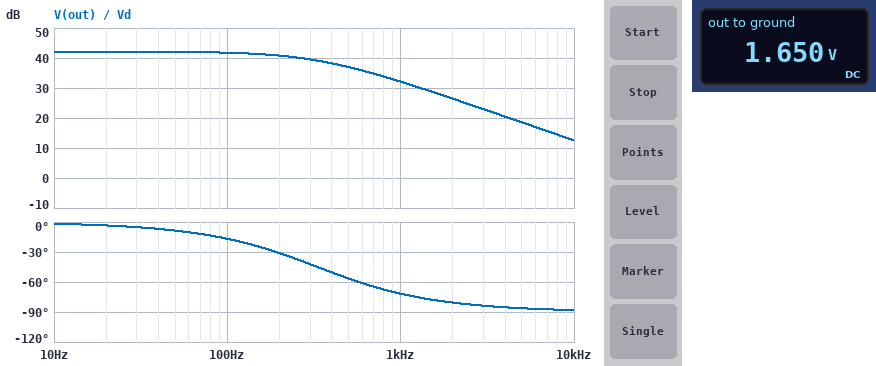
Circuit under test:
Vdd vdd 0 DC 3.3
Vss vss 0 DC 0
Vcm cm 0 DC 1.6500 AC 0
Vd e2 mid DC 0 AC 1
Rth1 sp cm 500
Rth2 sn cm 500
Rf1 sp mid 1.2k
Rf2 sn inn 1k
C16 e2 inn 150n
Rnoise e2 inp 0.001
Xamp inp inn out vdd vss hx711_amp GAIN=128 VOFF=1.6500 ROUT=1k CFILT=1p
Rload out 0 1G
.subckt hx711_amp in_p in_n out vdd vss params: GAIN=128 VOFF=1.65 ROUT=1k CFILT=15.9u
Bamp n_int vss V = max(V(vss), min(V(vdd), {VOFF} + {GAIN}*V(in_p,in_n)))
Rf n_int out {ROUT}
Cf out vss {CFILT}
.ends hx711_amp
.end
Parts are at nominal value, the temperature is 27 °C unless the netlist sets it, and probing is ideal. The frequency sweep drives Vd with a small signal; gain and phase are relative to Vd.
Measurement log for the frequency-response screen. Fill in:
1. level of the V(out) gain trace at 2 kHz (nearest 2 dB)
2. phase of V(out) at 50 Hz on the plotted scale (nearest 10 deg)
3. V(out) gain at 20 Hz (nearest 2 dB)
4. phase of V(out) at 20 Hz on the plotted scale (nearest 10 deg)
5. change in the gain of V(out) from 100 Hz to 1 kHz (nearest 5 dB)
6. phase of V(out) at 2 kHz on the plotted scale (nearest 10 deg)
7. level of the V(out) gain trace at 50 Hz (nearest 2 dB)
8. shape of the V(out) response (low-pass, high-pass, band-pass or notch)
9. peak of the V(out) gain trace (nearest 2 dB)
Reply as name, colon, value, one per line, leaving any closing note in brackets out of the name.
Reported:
level of the V(out) gain trace at 2 kHz: 26 dB
phase of V(out) at 50 Hz on the plotted scale: -10 deg
V(out) gain at 20 Hz: 42 dB
phase of V(out) at 20 Hz on the plotted scale: 0 deg
change in the gain of V(out) from 100 Hz to 1 kHz: -10 dB
phase of V(out) at 2 kHz on the plotted scale: -80 deg
level of the V(out) gain trace at 50 Hz: 42 dB
shape of the V(out) response: low-pass
peak of the V(out) gain trace: 42 dB
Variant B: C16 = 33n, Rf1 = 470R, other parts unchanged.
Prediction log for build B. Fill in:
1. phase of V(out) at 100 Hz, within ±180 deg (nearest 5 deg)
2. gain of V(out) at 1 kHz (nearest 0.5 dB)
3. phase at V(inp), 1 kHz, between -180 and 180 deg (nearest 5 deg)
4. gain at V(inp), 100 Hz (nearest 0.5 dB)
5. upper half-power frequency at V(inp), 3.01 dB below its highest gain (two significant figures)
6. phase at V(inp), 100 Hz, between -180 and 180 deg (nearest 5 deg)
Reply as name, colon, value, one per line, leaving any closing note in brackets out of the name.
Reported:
phase of V(out) at 100 Hz, within ±180 deg: -5 deg
gain of V(out) at 1 kHz: 41.0 dB
phase at V(inp), 1 kHz, between -180 and 180 deg: -10 deg
gain at V(inp), 100 Hz: 0 dB
upper half-power frequency at V(inp), 3.01 dB below its highest gain: 3.8 kHz
phase at V(inp), 100 Hz, between -180 and 180 deg: 0 deg
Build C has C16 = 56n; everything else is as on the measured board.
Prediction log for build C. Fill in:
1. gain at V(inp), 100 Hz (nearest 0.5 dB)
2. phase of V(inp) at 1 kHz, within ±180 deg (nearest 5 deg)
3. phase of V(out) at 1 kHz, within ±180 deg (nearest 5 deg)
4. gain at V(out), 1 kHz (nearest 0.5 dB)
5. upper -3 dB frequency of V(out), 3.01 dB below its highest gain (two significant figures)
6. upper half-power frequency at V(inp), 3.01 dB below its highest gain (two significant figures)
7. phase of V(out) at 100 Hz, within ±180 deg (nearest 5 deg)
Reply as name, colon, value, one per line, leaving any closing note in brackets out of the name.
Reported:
gain at V(inp), 100 Hz: 0 dB
phase of V(inp) at 1 kHz, within ±180 deg: -20 deg
phase of V(out) at 1 kHz, within ±180 deg: -50 deg
gain at V(out), 1 kHz: 38.5 dB
upper -3 dB frequency of V(out), 3.01 dB below its highest gain: 890 Hz
upper half-power frequency at V(inp), 3.01 dB below its highest gain: 1.2 kHz
phase of V(out) at 100 Hz, within ±180 deg: -5 deg
